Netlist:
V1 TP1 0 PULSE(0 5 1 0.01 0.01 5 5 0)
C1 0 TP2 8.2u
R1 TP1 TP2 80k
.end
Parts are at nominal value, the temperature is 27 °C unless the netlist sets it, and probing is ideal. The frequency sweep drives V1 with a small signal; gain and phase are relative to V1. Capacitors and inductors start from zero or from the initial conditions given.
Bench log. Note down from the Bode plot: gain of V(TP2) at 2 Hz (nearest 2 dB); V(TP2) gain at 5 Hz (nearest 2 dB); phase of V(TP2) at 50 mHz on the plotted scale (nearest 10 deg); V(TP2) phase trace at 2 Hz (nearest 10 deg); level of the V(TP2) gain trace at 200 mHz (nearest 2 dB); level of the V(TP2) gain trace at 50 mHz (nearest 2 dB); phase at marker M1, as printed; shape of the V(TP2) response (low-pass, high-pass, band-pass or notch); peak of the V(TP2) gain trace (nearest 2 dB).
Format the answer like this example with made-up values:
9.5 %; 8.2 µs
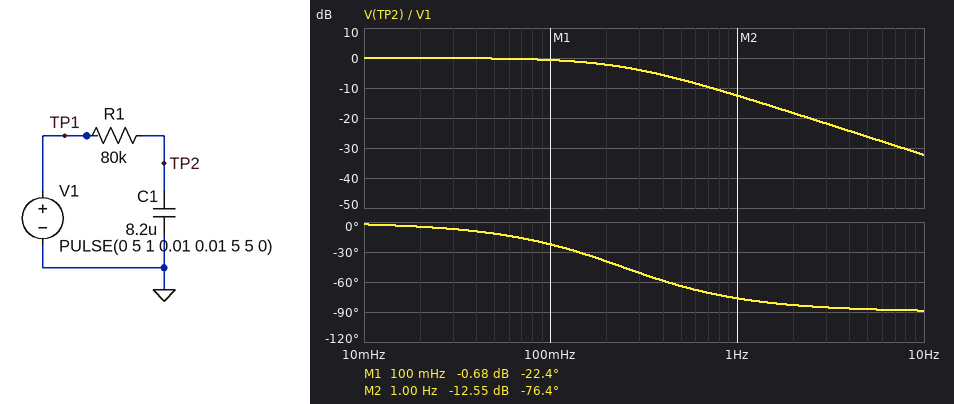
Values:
-18 dB; -26 dB; -10 deg; -80 deg; -2 dB; 0 dB; -22.4 deg; low-pass; 0 dB
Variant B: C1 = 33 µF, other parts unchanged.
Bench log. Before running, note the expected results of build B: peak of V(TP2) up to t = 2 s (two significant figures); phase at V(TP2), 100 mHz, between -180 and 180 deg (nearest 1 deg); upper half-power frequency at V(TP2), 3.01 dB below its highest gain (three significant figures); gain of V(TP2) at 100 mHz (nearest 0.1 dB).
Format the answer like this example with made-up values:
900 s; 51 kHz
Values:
1.6 V; -59 deg; 60.3 mHz; -5.7 dB
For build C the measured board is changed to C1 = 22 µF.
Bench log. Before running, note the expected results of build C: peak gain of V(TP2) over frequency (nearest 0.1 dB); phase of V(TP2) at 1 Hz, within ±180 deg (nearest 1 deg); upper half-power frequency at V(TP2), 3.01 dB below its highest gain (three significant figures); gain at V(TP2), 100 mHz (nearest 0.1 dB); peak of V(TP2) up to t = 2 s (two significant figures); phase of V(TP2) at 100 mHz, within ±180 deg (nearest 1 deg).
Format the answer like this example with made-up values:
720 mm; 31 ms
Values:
0 dB; -85 deg; 90.4 mHz; -3.5 dB; 2.2 V; -48 deg
